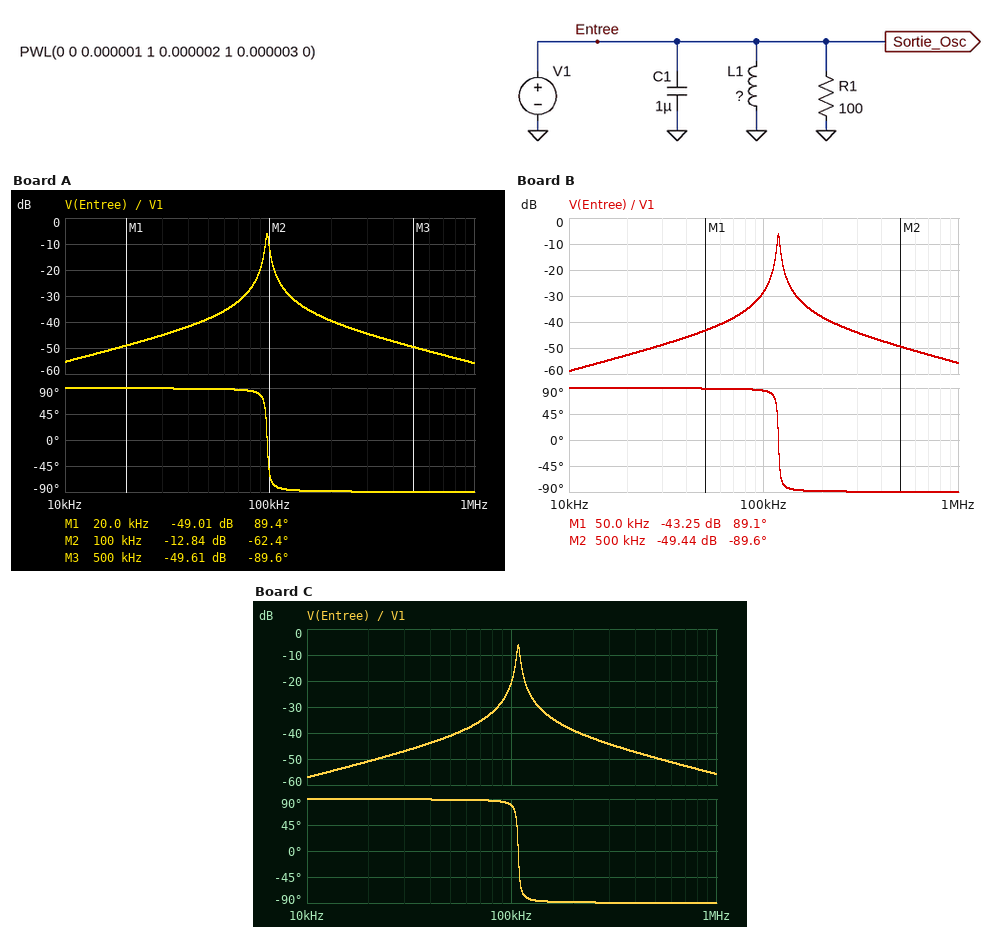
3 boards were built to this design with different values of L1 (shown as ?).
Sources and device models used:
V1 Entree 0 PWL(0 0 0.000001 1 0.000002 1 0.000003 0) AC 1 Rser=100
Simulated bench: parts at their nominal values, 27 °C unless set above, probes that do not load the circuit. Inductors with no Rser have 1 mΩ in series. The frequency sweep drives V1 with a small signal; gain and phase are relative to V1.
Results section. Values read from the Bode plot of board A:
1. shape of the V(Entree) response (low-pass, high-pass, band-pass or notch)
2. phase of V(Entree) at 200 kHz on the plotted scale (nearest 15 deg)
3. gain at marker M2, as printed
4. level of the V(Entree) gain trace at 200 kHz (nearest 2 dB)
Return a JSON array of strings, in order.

["band-pass", "-90 deg", "-12.84 dB", "-40 dB"]
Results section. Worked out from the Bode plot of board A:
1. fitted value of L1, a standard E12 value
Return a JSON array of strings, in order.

["2.7 µH"]
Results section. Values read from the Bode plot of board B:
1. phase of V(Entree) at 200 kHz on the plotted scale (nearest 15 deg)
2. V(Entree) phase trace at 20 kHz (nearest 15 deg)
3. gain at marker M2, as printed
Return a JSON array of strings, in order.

["-90 deg", "90 deg", "-49.44 dB"]
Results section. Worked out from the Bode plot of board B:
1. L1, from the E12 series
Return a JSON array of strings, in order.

["1.8 µH"]
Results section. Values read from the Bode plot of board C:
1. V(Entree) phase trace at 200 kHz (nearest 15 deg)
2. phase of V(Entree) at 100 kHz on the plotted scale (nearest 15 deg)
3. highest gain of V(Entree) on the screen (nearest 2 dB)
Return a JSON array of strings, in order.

["-90 deg", "75 deg", "-6 dB"]
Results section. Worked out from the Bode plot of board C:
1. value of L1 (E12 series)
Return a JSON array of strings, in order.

["2.2 µH"]
